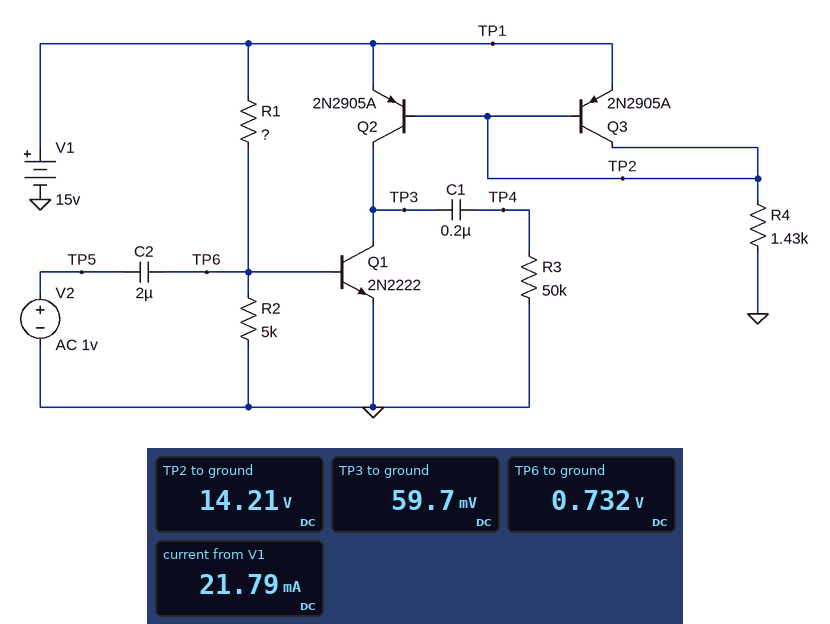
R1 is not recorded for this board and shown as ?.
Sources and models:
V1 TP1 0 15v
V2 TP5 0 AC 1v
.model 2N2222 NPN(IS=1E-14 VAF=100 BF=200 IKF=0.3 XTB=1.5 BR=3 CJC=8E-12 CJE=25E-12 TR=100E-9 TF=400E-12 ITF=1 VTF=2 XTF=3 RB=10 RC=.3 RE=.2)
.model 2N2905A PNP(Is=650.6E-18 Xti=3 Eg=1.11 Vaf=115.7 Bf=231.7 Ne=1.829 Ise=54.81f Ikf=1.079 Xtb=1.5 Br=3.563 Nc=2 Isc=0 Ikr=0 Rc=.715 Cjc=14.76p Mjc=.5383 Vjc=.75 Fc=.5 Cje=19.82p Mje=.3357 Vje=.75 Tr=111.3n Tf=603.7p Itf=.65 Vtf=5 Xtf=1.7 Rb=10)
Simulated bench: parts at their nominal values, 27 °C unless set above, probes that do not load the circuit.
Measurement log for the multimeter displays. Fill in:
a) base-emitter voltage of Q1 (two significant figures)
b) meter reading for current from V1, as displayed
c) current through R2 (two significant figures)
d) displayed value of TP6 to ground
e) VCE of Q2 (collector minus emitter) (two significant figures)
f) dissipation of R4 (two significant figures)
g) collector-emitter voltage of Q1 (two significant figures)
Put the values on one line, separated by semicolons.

730 mV; 21.79 mA; 150 µA; 0.732 V; -15 V; 140 mW; 60 mV
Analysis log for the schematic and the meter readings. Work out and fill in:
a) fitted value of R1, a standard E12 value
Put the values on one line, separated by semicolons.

18 kΩ
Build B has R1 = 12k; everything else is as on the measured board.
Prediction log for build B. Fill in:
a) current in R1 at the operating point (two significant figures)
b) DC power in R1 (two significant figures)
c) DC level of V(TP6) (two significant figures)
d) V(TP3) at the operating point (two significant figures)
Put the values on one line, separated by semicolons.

1.2 mA; 17 mW; 740 mV; 49 mV
